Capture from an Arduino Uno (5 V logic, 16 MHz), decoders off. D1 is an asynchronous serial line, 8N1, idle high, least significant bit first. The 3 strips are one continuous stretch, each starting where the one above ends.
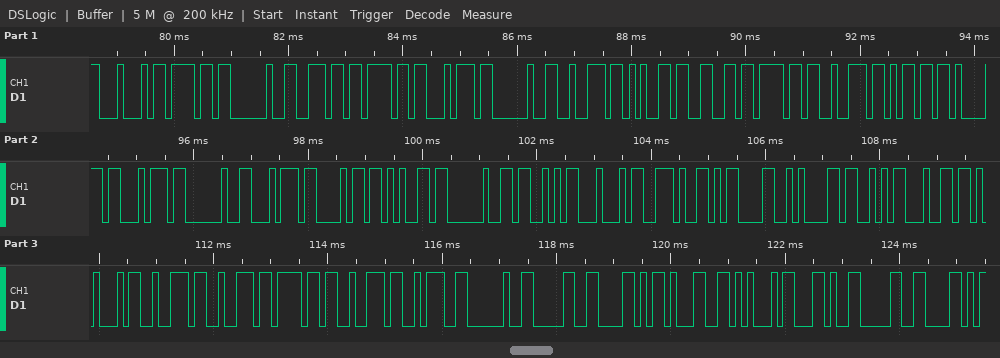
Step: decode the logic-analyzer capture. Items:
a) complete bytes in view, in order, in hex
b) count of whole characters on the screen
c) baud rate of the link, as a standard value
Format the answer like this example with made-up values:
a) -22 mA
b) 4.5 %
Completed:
a) 44 6F 20 6E 6F 74 20 72 65 66 6F 72 6D 61 74 20 74 68 65 20 53 44 2E 0D 0A 53 64 45 72 72 6F 72 3A 20 30 58 31 45 2C 30 58
b) 41
c) 9600 baud
